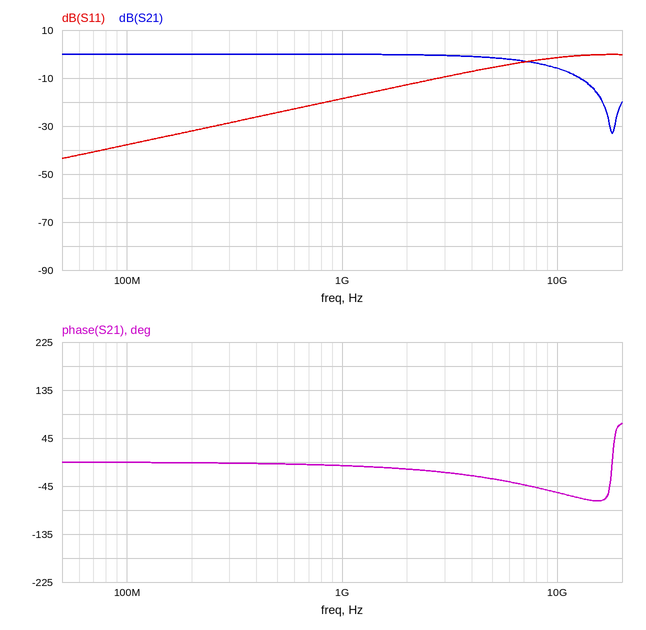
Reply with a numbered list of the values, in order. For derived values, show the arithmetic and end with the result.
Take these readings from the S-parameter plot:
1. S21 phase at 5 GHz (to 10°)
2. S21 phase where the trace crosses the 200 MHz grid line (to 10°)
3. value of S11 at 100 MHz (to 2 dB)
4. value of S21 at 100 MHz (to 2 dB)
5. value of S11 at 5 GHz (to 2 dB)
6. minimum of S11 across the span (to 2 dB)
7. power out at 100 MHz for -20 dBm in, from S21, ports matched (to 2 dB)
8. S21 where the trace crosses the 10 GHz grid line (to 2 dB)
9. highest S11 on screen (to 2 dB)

1. -30°
2. 0°
3. -38 dB
4. 0 dB
5. -6 dB
6. -44 dB
7. -20 dBm + (0 dB) = -20 dBm
8. -6 dB
9. 0 dB
